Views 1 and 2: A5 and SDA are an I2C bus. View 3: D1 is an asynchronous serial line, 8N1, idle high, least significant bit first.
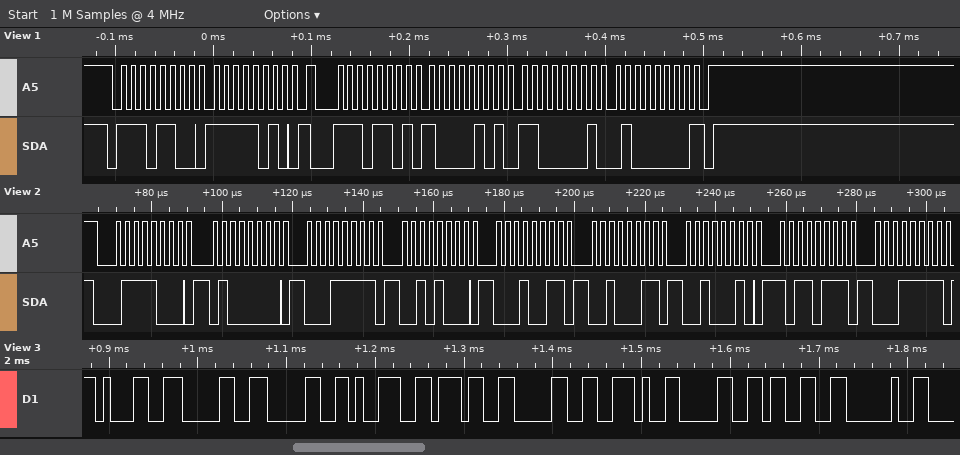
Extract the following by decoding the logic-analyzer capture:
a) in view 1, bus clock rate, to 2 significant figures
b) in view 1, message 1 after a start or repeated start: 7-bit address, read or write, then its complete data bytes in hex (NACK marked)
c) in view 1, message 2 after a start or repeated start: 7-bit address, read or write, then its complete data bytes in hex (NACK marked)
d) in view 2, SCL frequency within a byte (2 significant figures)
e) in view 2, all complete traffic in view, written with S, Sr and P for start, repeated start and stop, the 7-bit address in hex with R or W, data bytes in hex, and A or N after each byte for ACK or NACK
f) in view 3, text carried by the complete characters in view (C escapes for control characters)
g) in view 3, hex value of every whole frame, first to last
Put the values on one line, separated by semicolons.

100 kHz; 0x76 write: FA; 0x76 read: 85 C1 40 NACK; 400 kHz; S 3CW A 40 A 1F A 28 A 13 A 23 A 22 A B7 A 1F A; "100970.03 "; 31 30 30 39 37 30 2E 30 33 20
